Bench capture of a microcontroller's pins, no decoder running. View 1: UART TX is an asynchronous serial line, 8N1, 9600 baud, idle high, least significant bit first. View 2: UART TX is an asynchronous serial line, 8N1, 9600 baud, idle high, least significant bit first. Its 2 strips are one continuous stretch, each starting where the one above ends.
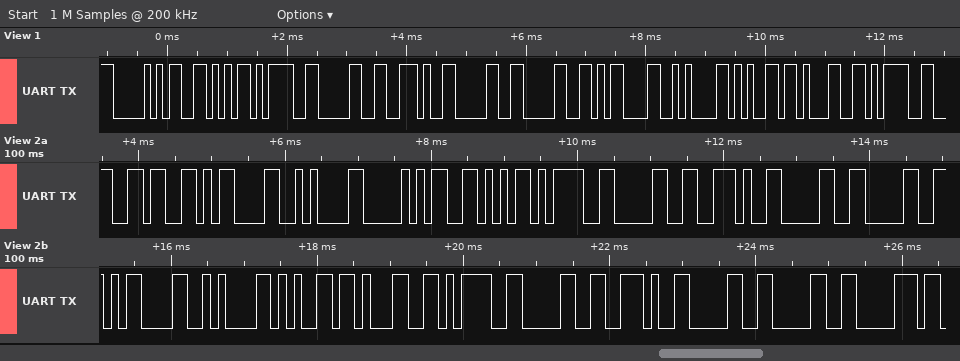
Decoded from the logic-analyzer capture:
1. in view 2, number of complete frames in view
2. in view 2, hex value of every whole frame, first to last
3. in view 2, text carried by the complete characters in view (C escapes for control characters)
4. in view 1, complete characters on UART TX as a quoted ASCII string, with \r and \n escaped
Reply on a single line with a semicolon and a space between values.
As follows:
20; 36 0D 0A 50 56 3D 30 2E 30 30 0D 0A 65 31 3D 30 2E 30 30 70; "6\r\nPV=0.00\r\ne1=0.00p"; "PV=0.00\r\ne1="
